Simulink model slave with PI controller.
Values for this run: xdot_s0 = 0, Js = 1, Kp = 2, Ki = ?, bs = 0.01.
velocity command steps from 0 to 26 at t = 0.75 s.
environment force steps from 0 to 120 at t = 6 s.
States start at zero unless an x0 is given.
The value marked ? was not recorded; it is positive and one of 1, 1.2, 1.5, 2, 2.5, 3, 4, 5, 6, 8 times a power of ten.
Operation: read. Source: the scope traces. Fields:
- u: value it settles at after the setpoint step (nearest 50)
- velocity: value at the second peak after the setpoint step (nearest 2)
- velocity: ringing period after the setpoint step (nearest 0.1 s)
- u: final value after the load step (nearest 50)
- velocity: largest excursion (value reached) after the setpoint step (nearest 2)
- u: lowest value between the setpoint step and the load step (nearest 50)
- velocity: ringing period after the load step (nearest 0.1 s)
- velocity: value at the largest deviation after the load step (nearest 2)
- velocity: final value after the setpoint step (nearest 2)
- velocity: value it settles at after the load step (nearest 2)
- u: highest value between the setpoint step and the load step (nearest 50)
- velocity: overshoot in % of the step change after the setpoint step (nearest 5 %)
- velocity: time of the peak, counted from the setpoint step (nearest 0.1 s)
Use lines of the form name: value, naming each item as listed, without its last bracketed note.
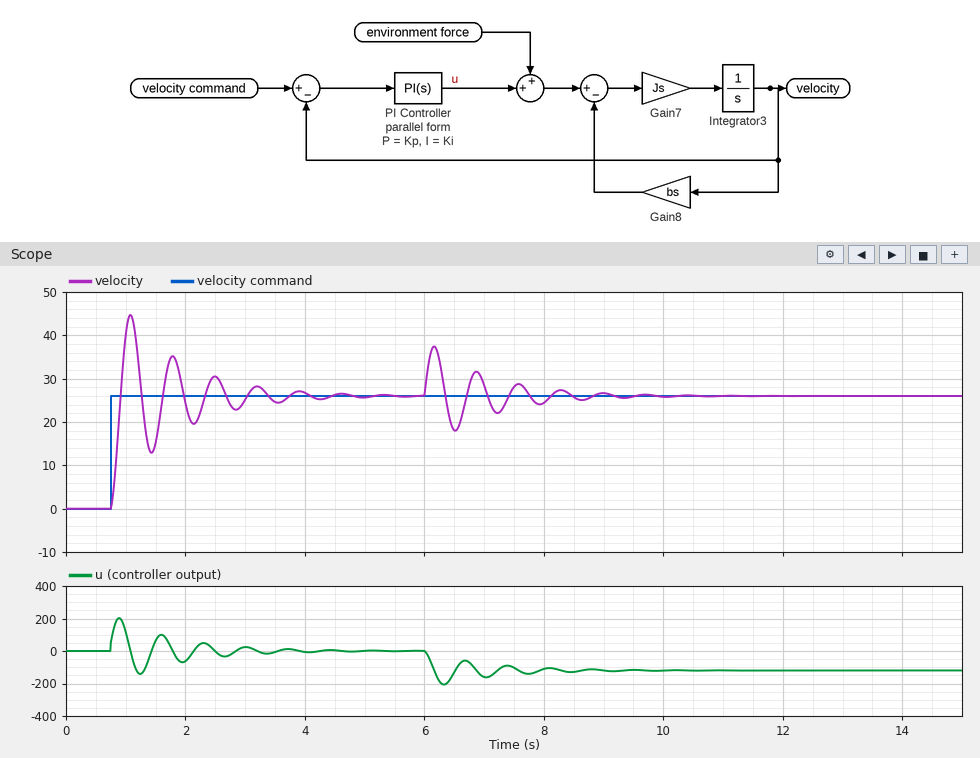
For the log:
u: value it settles at after the setpoint step: 0
velocity: value at the second peak after the setpoint step: 36
velocity: ringing period after the setpoint step: 0.7 s
u: final value after the load step: -100
velocity: largest excursion (value reached) after the setpoint step: 44
u: lowest value between the setpoint step and the load step: -150
velocity: ringing period after the load step: 0.7 s
velocity: value at the largest deviation after the load step: 38
velocity: final value after the setpoint step: 26
velocity: value it settles at after the load step: 26
u: highest value between the setpoint step and the load step: 200
velocity: overshoot in % of the step change after the setpoint step: 70 %
velocity: time of the peak, counted from the setpoint step: 0.3 s
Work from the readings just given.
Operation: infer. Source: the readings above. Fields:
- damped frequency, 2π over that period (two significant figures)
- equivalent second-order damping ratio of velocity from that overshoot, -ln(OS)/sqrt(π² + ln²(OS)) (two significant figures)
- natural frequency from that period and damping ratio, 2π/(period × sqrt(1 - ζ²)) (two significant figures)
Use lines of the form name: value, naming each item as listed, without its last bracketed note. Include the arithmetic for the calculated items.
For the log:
damped frequency, 2π over that period: 2π / 0.7 = 9.0 rad/s
equivalent second-order damping ratio of velocity from that overshoot, -ln(OS)/sqrt(π² + ln²(OS)): ln(0.7) = -0.357; 0.357 / sqrt(9.870 + 0.127) = 0.11
natural frequency from that period and damping ratio, 2π/(period × sqrt(1 - ζ²)): 2π / (0.7 × sqrt(1 - 0.11²)) = 9.0 rad/s
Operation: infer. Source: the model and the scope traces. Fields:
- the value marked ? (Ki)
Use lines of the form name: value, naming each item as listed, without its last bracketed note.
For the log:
the value marked ?: 80
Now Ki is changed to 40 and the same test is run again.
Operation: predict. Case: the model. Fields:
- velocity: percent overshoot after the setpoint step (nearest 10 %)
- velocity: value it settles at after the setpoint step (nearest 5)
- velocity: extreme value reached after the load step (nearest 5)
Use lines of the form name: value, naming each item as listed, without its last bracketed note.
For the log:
velocity: percent overshoot after the setpoint step: 60 %
velocity: value it settles at after the setpoint step: 25
velocity: extreme value reached after the load step: 40
